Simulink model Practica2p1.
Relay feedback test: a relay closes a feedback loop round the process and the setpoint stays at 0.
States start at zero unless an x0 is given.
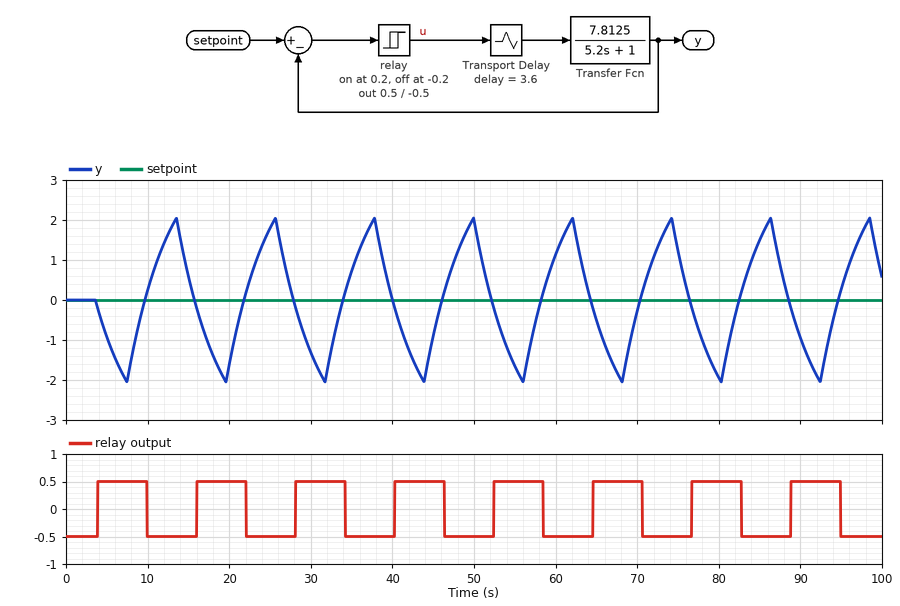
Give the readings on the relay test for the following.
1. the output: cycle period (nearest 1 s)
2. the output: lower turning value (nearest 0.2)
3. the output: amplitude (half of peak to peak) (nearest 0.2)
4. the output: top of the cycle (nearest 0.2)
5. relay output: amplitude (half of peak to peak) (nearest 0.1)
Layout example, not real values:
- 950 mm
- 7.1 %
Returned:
- 12 s
- -2.0
- 2.0
- 2.0
- 0.5
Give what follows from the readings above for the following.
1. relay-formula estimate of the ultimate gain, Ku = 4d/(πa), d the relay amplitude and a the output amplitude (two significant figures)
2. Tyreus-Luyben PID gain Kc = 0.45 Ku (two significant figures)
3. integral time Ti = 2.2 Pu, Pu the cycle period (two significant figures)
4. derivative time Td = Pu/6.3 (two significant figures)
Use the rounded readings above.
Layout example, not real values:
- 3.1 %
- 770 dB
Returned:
- 0.32
- 0.14
- 26 s
- 1.9 s
